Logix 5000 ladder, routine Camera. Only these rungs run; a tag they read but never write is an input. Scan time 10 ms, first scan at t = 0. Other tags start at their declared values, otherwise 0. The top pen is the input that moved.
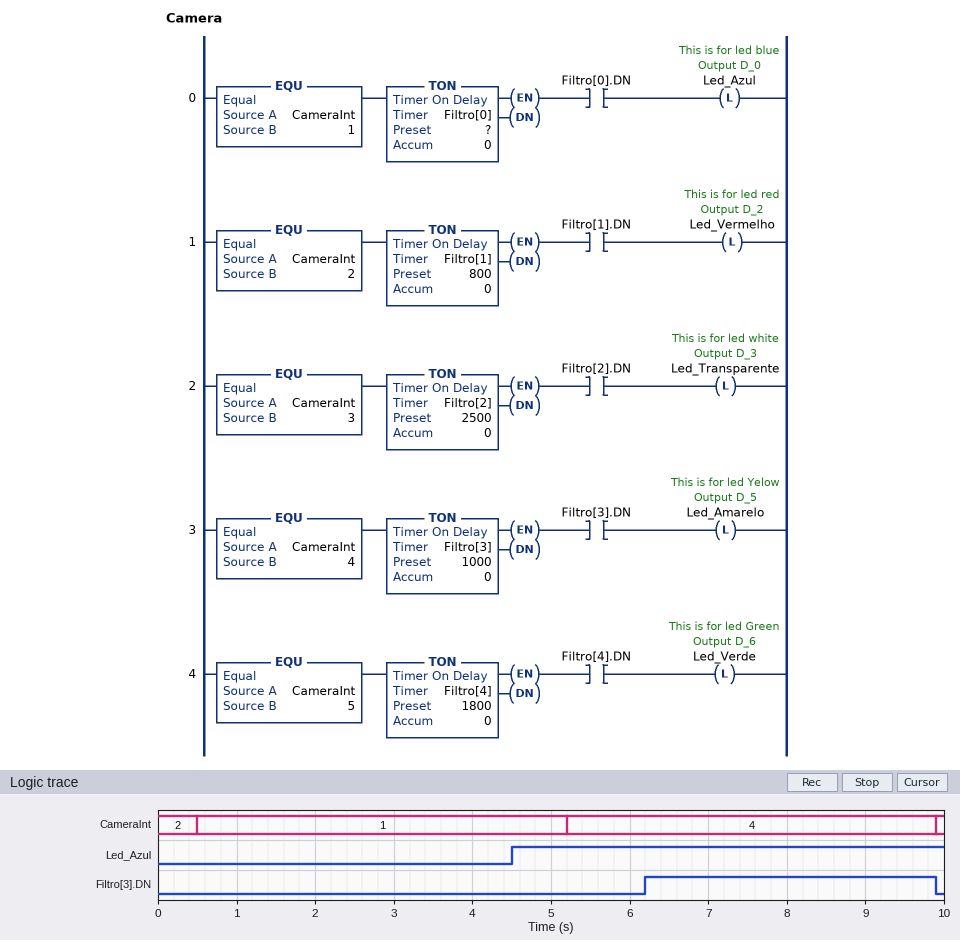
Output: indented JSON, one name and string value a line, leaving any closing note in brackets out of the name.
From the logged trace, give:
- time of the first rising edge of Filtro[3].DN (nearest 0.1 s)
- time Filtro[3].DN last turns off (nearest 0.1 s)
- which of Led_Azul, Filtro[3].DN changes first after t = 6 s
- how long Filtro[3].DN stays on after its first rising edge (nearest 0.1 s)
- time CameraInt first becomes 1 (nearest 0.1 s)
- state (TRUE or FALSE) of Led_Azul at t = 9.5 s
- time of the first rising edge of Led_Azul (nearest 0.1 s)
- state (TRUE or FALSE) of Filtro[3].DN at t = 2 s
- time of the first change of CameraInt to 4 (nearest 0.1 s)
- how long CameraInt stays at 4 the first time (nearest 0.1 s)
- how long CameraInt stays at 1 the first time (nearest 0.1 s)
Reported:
{
  "time of the first rising edge of Filtro[3].DN": "6.2 s",
  "time Filtro[3].DN last turns off": "9.9 s",
  "which of Led_Azul, Filtro[3].DN changes first after t = 6 s": "Filtro[3].DN",
  "how long Filtro[3].DN stays on after its first rising edge": "3.7 s",
  "time CameraInt first becomes 1": "0.5 s",
  "state (TRUE or FALSE) of Led_Azul at t = 9.5 s": "TRUE",
  "time of the first rising edge of Led_Azul": "4.5 s",
  "state (TRUE or FALSE) of Filtro[3].DN at t = 2 s": "FALSE",
  "time of the first change of CameraInt to 4": "5.2 s",
  "how long CameraInt stays at 4 the first time": "4.7 s",
  "how long CameraInt stays at 1 the first time": "4.7 s"
}
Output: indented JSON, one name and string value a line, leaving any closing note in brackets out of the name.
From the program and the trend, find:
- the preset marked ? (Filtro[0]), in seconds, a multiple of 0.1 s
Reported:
{
  "the preset marked ? (Filtro[0]), in seconds, a multiple of 0.1 s": "4.0 s"
}
